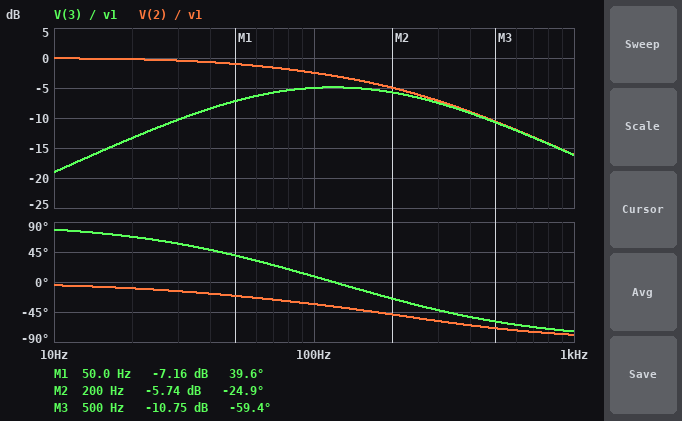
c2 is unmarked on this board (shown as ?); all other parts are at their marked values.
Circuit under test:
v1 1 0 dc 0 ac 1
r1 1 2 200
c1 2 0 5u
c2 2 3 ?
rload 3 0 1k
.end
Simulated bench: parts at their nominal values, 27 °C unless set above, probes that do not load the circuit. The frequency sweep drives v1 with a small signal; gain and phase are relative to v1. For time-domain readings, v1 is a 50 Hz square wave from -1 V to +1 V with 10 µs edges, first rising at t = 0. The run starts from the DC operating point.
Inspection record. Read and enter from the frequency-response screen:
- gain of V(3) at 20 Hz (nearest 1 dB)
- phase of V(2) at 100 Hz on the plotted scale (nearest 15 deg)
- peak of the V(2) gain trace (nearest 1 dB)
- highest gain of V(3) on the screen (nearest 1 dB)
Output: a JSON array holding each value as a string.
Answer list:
["-13 dB", "-30 deg", "0 dB", "-5 dB"]
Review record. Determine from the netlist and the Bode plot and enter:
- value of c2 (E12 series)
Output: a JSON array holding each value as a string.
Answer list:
["1.8 µF"]
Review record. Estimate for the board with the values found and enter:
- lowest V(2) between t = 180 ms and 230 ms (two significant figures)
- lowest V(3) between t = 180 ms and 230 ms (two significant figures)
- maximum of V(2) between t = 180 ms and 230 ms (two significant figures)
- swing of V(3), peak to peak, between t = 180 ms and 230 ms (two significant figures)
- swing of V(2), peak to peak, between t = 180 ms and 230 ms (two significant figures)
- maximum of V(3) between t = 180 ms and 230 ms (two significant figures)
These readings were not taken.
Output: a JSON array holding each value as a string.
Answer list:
["-990 mV", "-860 mV", "990 mV", "1.7 V", "2.0 V", "860 mV"]
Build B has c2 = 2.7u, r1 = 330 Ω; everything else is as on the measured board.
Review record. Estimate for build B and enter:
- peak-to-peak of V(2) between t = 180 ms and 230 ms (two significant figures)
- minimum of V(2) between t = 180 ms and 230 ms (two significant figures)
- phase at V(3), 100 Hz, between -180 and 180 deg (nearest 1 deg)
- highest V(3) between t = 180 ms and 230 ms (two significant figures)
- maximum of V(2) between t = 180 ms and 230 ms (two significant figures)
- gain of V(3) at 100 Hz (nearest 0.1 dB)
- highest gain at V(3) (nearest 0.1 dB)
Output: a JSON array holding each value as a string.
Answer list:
["1.8 V", "-920 mV", "-13 deg", "720 mV", "920 mV", "-6.0 dB", "-5.8 dB"]
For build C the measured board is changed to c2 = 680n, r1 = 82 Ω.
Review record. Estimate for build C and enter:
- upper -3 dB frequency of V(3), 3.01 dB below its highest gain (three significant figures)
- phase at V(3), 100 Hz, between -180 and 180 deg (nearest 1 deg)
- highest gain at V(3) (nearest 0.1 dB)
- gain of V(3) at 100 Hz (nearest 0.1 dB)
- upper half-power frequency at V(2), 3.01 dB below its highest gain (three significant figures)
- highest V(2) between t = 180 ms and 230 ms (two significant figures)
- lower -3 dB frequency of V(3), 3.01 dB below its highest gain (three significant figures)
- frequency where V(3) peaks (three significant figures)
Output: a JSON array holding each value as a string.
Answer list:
["772 Hz", "51 deg", "-4.5 dB", "-8.6 dB", "350 Hz", "1.0 V", "118 Hz", "301 Hz"]
